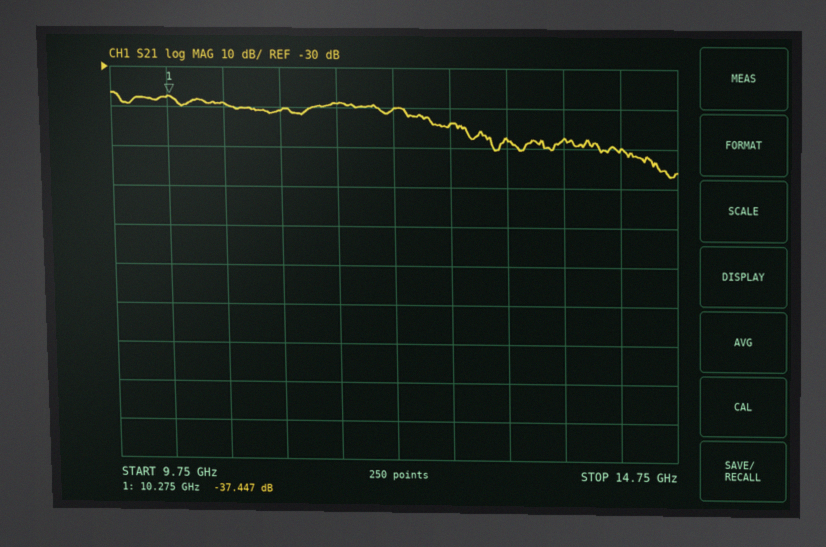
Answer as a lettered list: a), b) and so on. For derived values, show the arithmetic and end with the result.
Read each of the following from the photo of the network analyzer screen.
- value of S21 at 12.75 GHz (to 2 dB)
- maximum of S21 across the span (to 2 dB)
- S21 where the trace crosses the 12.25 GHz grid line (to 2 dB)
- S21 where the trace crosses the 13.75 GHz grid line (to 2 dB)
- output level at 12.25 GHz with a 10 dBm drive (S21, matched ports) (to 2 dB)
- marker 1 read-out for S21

a) -44 dB
b) -36 dB
c) -40 dB
d) -48 dB
e) 10 dBm + (-40 dB) = -30 dBm
f) -37.447 dB
